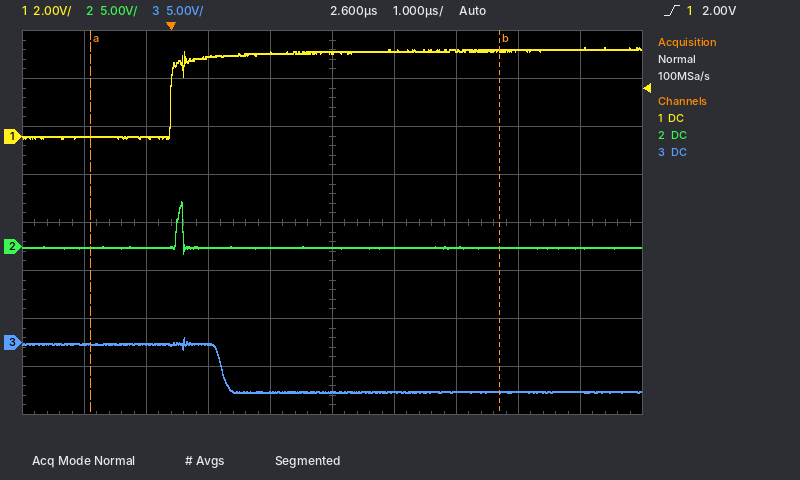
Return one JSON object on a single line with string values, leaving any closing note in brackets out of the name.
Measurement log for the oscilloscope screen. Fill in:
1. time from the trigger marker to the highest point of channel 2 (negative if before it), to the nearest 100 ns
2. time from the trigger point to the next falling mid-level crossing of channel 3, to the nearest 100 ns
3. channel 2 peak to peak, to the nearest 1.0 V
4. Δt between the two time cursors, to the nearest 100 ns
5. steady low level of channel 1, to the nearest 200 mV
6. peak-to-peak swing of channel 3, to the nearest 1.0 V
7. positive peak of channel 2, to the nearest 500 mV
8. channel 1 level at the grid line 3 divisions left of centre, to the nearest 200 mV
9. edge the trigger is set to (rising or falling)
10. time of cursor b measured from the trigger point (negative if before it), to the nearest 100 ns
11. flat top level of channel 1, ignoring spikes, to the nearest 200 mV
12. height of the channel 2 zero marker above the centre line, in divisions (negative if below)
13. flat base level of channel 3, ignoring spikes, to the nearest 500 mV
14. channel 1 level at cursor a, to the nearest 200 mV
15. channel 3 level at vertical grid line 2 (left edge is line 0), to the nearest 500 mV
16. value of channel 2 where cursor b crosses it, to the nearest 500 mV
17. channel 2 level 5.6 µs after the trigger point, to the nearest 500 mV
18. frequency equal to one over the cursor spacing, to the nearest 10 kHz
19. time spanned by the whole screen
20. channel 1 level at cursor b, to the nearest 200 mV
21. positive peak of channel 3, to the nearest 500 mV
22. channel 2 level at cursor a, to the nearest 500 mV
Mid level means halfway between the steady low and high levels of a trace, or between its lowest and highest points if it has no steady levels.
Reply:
{"time from the trigger marker to the highest point of channel 2 (negative if before it), to the nearest 100 ns": "+200 ns", "time from the trigger point to the next falling mid-level crossing of channel 3, to the nearest 100 ns": "800 ns", "channel 2 peak to peak, to the nearest 1.0 V": "5.0 V", "Δt between the two time cursors, to the nearest 100 ns": "6.6 µs", "steady low level of channel 1, to the nearest 200 mV": "0.0 V", "peak-to-peak swing of channel 3, to the nearest 1.0 V": "6.0 V", "positive peak of channel 2, to the nearest 500 mV": "4.5 V", "channel 1 level at the grid line 3 divisions left of centre, to the nearest 200 mV": "0.0 V", "edge the trigger is set to": "rising", "time of cursor b measured from the trigger point (negative if before it), to the nearest 100 ns": "+5.3 µs", "flat top level of channel 1, ignoring spikes, to the nearest 200 mV": "3.6 V", "height of the channel 2 zero marker above the centre line, in divisions": "-0.5 div", "flat base level of channel 3, ignoring spikes, to the nearest 500 mV": "-5.0 V", "channel 1 level at cursor a, to the nearest 200 mV": "0.0 V", "channel 3 level at vertical grid line 2 (left edge is line 0), to the nearest 500 mV": "0.0 V", "value of channel 2 where cursor b crosses it, to the nearest 500 mV": "0.0 V", "channel 2 level 5.6 µs after the trigger point, to the nearest 500 mV": "0.0 V", "frequency equal to one over the cursor spacing, to the nearest 10 kHz": "150 kHz", "time spanned by the whole screen": "10 µs", "channel 1 level at cursor b, to the nearest 200 mV": "3.6 V", "positive peak of channel 3, to the nearest 500 mV": "500 mV", "channel 2 level at cursor a, to the nearest 500 mV": "0.0 V"}
